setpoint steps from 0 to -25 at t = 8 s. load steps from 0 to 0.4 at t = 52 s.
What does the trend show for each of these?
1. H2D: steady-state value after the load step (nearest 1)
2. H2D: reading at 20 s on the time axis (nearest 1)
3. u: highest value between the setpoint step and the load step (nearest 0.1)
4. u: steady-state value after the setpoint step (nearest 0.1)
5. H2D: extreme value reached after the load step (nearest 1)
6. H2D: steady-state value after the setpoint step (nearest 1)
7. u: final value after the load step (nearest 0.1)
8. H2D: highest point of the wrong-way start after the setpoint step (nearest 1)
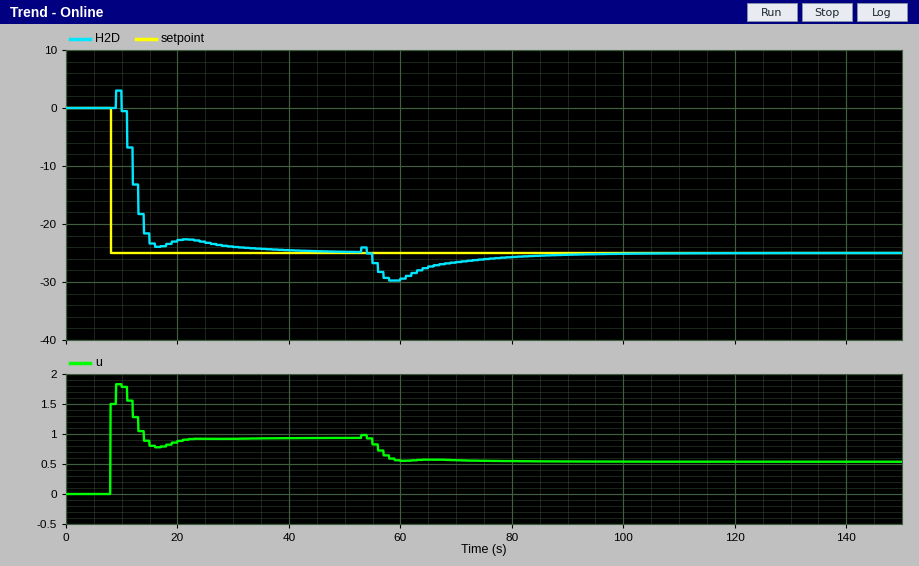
-25
-23
1.8
0.9
-30
-25
0.5
3
